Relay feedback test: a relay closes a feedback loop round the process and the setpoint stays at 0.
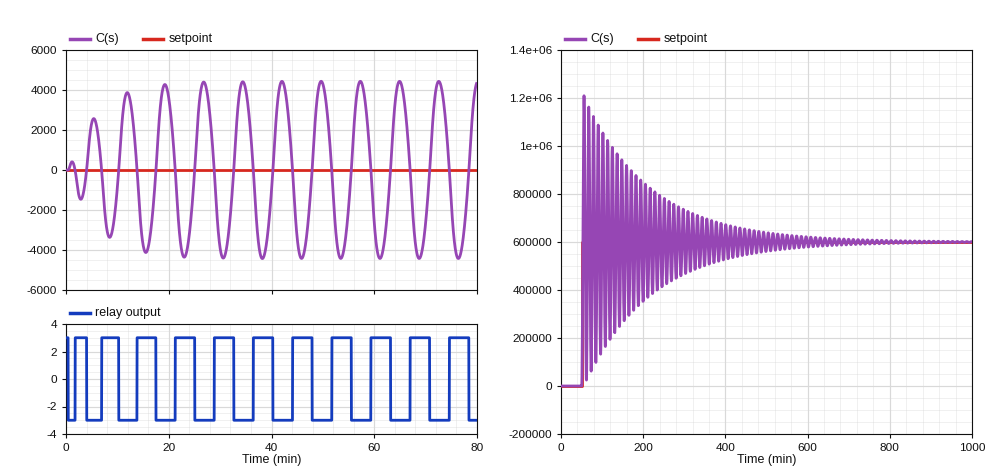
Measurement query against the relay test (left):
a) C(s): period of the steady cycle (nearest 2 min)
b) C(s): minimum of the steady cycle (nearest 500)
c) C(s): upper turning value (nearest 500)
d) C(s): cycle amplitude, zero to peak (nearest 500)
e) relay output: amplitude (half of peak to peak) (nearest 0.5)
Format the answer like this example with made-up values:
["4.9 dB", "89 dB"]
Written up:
["8 min", "-4500", "4500", "4500", "3.0"]
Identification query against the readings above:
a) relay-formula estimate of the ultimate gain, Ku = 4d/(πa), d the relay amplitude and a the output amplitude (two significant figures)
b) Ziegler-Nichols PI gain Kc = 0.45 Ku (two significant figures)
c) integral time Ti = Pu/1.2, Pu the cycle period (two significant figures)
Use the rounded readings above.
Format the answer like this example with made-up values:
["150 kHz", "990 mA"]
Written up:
["0.00085", "0.00038", "6.7 min"]
